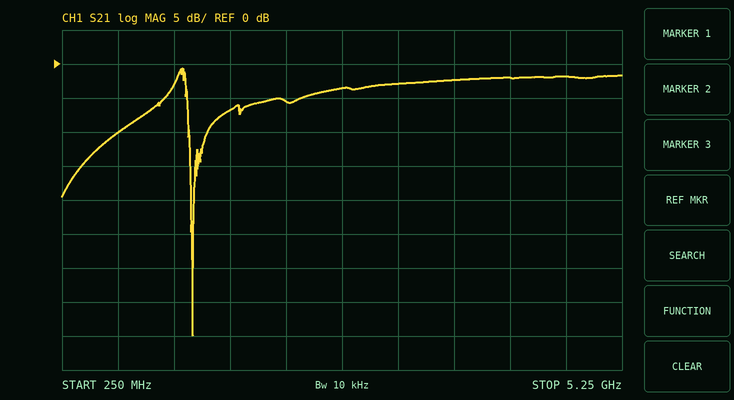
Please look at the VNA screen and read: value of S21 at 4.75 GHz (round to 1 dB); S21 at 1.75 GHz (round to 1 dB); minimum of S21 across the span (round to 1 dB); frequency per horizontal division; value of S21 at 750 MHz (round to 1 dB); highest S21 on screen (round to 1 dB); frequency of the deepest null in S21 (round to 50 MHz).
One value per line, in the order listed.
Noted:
-2 dB
-7 dB
-40 dB
500 MHz
-10 dB
-1 dB
1.40 GHz
